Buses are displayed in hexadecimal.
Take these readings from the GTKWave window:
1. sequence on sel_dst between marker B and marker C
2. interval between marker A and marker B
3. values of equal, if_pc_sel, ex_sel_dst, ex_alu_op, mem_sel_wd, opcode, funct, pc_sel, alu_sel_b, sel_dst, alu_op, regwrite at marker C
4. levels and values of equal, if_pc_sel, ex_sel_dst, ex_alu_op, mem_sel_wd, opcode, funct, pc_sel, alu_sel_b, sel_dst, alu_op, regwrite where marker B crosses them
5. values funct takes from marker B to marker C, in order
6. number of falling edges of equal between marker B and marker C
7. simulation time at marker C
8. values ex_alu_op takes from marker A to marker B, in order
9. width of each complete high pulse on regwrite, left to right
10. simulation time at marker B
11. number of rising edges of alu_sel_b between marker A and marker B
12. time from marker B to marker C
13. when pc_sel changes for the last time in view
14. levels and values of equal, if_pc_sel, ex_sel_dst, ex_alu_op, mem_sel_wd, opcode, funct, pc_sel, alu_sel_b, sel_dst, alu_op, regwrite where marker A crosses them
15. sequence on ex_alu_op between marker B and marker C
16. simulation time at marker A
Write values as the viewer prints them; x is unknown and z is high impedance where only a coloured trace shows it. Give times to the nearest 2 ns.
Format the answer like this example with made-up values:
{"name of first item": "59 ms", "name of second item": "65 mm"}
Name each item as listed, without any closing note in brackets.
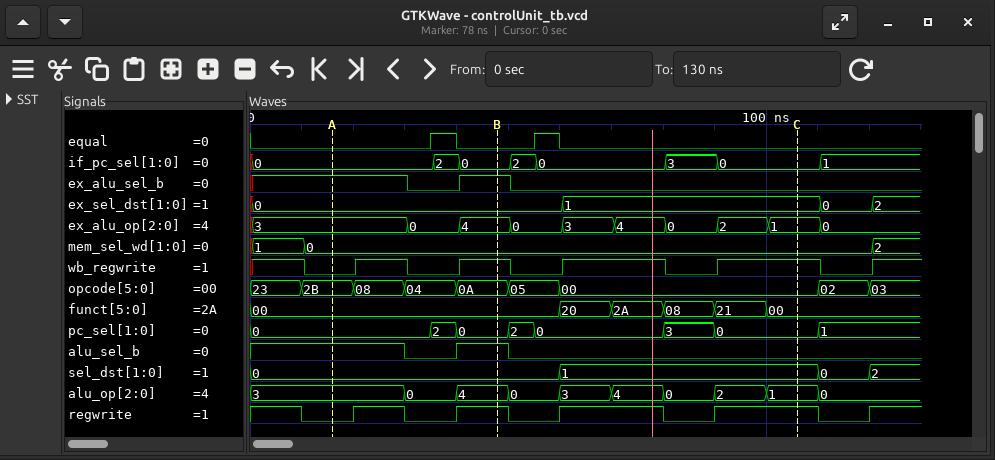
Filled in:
{"sequence on sel_dst between marker B and marker C": "0, 1", "interval between marker A and marker B": "32 ns", "values of equal, if_pc_sel, ex_sel_dst, ex_alu_op, mem_sel_wd, opcode, funct, pc_sel, alu_sel_b, sel_dst, alu_op, regwrite at marker C": "equal=0, if_pc_sel=0, ex_sel_dst=1, ex_alu_op=1, mem_sel_wd=0, opcode=00, funct=00, pc_sel=0, alu_sel_b=0, sel_dst=1, alu_op=1, regwrite=1", "levels and values of equal, if_pc_sel, ex_sel_dst, ex_alu_op, mem_sel_wd, opcode, funct, pc_sel, alu_sel_b, sel_dst, alu_op, regwrite where marker B crosses them": "equal=0, if_pc_sel=0, ex_sel_dst=0, ex_alu_op=4, mem_sel_wd=0, opcode=0A, funct=00, pc_sel=0, alu_sel_b=1, sel_dst=0, alu_op=4, regwrite=1", "values funct takes from marker B to marker C, in order": "00, 20, 2A, 08, 21, 00", "number of falling edges of equal between marker B and marker C": "1", "simulation time at marker C": "106 ns", "values ex_alu_op takes from marker A to marker B, in order": "3, 0, 4", "width of each complete high pulse on regwrite, left to right": "10 ns, 10 ns, 20 ns, 20 ns", "simulation time at marker B": "48 ns", "number of rising edges of alu_sel_b between marker A and marker B": "1", "time from marker B to marker C": "58 ns", "when pc_sel changes for the last time in view": "110 ns", "levels and values of equal, if_pc_sel, ex_sel_dst, ex_alu_op, mem_sel_wd, opcode, funct, pc_sel, alu_sel_b, sel_dst, alu_op, regwrite where marker A crosses them": "equal=0, if_pc_sel=0, ex_sel_dst=0, ex_alu_op=3, mem_sel_wd=0, opcode=2B, funct=00, pc_sel=0, alu_sel_b=1, sel_dst=0, alu_op=3, regwrite=0", "sequence on ex_alu_op between marker B and marker C": "4, 0, 3, 4, 0, 2, 1", "simulation time at marker A": "16 ns"}
